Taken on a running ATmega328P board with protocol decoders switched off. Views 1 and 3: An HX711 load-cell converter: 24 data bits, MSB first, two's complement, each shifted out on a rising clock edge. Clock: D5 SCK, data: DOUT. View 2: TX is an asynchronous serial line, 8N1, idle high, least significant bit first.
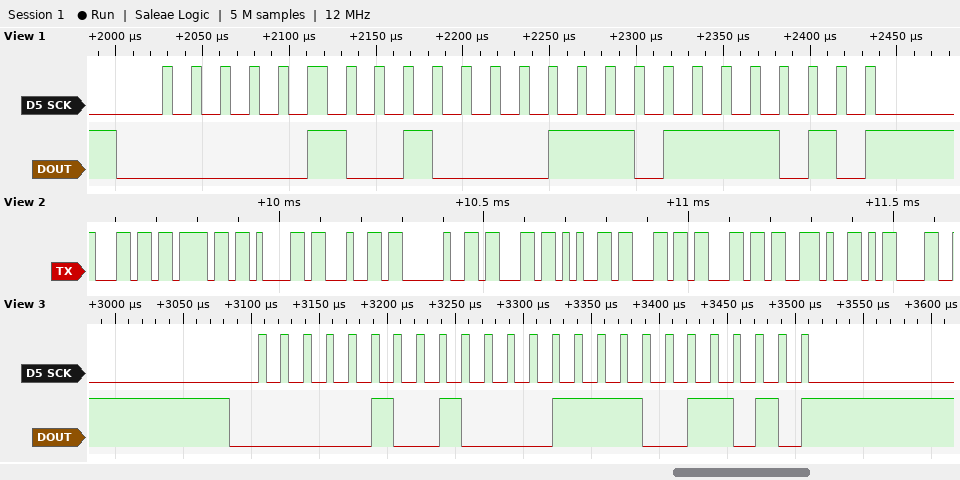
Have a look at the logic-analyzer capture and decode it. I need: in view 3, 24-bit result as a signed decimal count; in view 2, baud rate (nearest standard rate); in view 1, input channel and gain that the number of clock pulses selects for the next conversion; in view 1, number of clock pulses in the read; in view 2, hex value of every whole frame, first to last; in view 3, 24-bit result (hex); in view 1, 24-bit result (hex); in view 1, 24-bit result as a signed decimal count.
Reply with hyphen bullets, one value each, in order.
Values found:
- 296858
- 57600 baud
- channel A, gain 128
- 25
- 0x6C 0x6F 0x61 0x64 0x20 0x63 0x65 0x6C 0x6C 0x2E 0x0D
- 0x04879A
- 0x04877A
- 296826
